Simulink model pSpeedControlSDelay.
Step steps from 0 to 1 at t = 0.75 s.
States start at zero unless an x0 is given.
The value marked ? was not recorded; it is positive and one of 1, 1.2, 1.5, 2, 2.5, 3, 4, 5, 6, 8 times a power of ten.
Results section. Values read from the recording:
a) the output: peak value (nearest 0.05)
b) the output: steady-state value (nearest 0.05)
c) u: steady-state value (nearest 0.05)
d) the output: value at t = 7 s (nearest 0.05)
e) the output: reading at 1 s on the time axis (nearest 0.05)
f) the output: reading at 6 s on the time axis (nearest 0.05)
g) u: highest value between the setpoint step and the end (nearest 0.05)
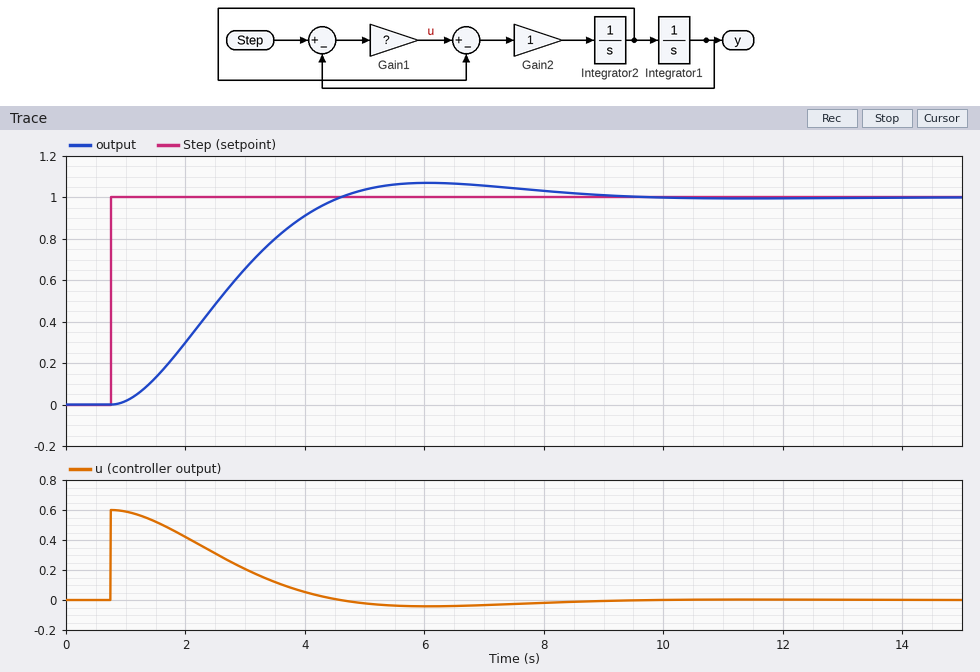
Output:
1.05
1.00
0.00
1.05
0.00
1.05
0.60
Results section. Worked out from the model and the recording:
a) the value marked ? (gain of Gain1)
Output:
0.6
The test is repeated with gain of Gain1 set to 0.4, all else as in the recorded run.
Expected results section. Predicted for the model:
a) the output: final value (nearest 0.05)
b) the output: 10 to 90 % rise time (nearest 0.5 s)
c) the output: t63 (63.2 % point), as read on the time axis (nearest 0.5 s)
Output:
1.00
4.0 s
3.5 s
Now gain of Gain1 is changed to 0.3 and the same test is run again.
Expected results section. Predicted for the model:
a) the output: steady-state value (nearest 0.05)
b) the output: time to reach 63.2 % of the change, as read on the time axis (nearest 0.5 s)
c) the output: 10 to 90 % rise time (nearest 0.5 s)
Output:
1.00
4.5 s
5.5 s
